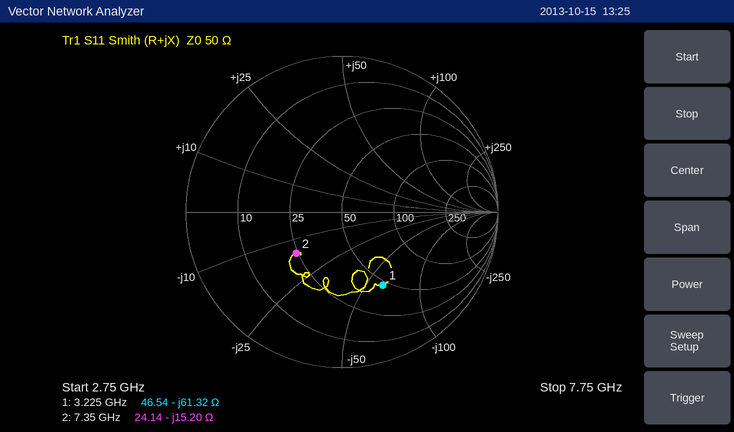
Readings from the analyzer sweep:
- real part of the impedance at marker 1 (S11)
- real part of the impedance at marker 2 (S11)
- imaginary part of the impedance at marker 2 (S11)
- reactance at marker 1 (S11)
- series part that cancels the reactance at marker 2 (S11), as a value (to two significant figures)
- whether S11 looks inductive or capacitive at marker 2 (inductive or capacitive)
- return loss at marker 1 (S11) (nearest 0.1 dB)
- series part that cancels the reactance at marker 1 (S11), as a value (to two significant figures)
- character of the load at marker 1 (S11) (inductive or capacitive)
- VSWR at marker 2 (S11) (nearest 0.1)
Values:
46.54 Ω
24.14 Ω
-15.20 Ω
-61.32 Ω
330 pH
capacitive
5.4 dB
3.0 nH
capacitive
2.3
